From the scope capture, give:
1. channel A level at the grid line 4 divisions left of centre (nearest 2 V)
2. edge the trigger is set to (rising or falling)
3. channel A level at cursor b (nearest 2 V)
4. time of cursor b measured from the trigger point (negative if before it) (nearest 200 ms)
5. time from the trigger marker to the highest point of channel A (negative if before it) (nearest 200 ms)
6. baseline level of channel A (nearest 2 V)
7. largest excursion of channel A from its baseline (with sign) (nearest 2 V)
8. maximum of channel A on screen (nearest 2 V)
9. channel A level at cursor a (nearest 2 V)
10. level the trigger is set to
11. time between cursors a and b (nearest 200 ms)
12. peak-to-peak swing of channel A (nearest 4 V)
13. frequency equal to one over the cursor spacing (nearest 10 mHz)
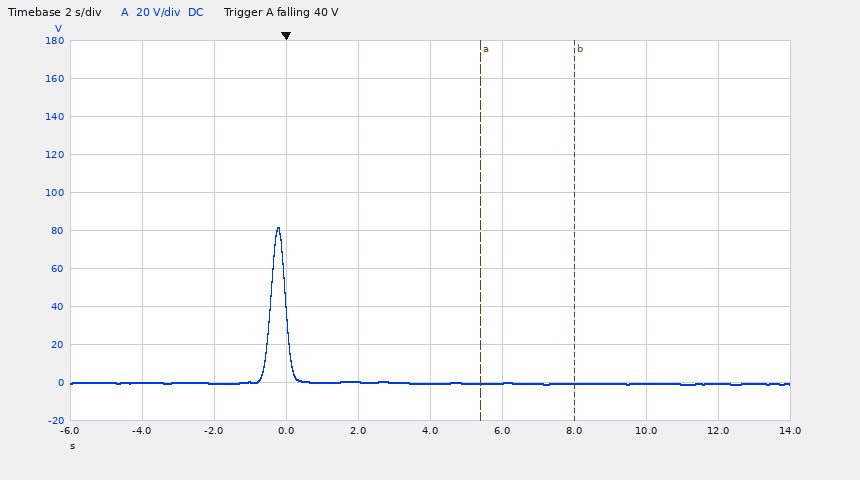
0 V
falling
0 V
+8.0 s
-200 ms
0 V
+82 V
82 V
0 V
40 V
2.6 s
84 V
380 mHz
